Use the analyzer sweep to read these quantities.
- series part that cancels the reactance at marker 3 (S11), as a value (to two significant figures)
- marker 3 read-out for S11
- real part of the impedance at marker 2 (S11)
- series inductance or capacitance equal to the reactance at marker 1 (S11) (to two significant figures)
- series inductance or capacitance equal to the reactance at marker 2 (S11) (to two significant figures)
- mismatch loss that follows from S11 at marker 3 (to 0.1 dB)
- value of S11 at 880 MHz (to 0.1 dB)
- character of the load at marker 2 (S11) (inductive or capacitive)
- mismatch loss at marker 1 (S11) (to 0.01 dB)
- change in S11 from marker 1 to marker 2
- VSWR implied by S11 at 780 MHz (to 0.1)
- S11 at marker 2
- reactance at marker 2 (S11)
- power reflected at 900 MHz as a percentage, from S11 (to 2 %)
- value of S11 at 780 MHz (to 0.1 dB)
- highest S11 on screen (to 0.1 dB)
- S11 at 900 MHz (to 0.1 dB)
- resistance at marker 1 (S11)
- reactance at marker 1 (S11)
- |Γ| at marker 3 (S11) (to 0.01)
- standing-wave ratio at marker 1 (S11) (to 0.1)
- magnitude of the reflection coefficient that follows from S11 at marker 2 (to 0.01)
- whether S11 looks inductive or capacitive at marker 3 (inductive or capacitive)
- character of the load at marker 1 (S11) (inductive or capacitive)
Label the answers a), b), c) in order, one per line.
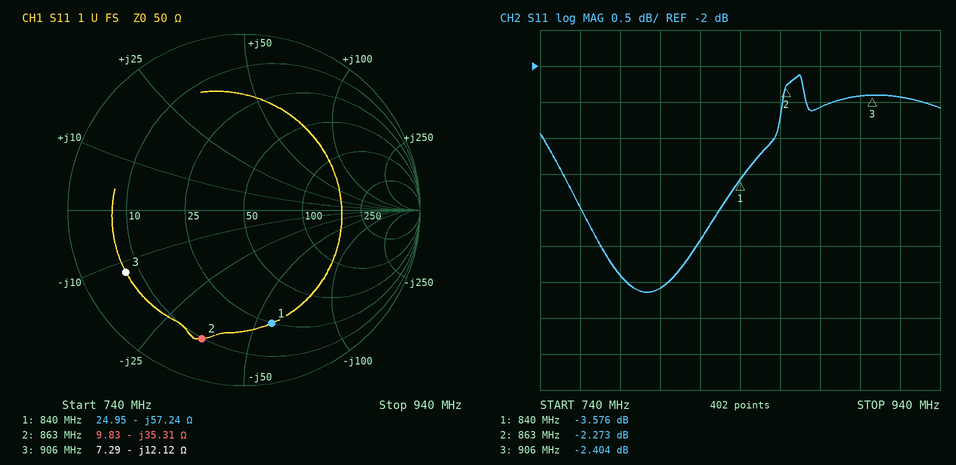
a) 2.1 nH
b) -2.404 dB
c) 9.83 Ω
d) 3.3 pF
e) 5.2 pF
f) 3.7 dB
g) -2.6 dB
h) capacitive
i) 2.51 dB
j) 1.303 dB
k) 3.6
l) -2.273 dB
m) -35.31 Ω
n) 58 %
o) -4.9 dB
p) -2.1 dB
q) -2.4 dB
r) 24.95 Ω
s) -57.24 Ω
t) 0.76
u) 4.9
v) 0.77
w) capacitive
x) capacitive
